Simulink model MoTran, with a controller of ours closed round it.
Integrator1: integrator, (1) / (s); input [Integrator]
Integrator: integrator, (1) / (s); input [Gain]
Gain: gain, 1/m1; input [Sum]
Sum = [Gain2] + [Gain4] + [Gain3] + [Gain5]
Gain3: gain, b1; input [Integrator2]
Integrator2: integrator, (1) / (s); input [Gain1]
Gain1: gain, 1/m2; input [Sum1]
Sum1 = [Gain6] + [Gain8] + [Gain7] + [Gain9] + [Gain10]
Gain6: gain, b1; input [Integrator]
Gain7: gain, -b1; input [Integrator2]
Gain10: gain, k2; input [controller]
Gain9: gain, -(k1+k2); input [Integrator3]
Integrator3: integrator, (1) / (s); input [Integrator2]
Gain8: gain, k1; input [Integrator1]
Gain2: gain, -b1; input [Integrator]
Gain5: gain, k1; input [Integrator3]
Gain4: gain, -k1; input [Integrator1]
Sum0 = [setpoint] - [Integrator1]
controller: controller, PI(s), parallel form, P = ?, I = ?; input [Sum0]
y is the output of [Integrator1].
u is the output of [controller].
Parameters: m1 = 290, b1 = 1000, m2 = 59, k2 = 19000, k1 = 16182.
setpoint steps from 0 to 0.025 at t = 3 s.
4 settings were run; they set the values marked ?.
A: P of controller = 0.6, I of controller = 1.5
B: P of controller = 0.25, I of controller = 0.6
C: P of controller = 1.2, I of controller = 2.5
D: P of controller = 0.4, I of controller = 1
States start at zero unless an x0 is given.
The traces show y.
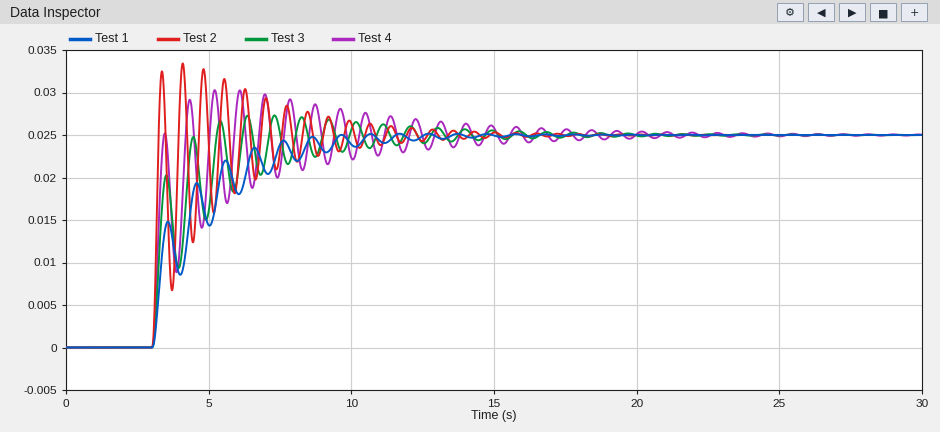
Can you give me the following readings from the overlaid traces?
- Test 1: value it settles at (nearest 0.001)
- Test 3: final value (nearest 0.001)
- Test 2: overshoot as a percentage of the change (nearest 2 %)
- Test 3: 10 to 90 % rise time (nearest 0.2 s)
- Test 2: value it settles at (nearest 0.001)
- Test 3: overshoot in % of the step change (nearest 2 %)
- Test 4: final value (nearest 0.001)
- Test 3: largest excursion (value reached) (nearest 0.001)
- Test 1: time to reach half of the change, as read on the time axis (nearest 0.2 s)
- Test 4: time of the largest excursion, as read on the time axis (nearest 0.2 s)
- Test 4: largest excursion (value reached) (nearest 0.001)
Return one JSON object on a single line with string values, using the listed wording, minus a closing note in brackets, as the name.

{"Test 1: value it settles at": "0.025", "Test 3: final value": "0.025", "Test 2: overshoot as a percentage of the change": "34 %", "Test 3: 10 to 90 % rise time": "1.2 s", "Test 2: value it settles at": "0.025", "Test 3: overshoot in % of the step change": "10 %", "Test 4: final value": "0.025", "Test 3: largest excursion (value reached)": "0.027", "Test 1: time to reach half of the change, as read on the time axis": "3.4 s", "Test 4: time of the largest excursion, as read on the time axis": "5.2 s", "Test 4: largest excursion (value reached)": "0.030"}
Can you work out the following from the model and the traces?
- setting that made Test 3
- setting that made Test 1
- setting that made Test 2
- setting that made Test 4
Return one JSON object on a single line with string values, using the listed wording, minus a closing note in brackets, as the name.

{"setting that made Test 3": "D", "setting that made Test 1": "B", "setting that made Test 2": "C", "setting that made Test 4": "A"}
